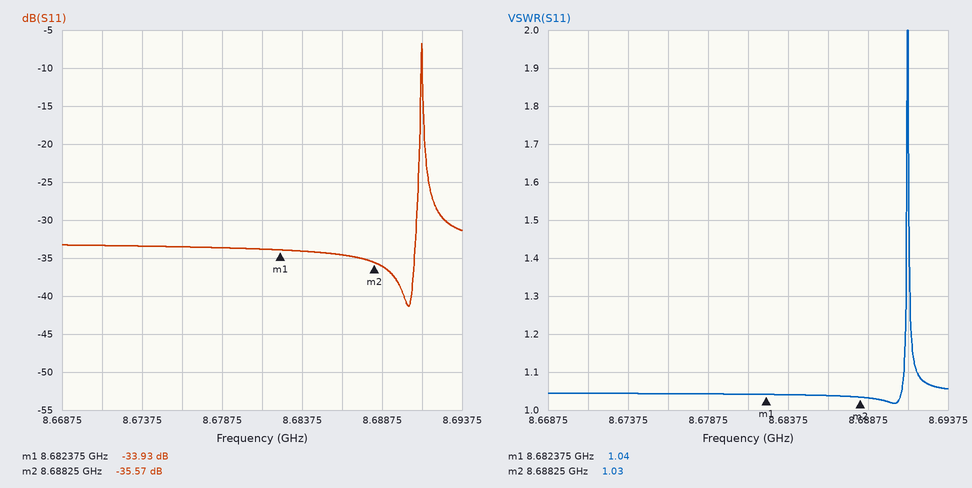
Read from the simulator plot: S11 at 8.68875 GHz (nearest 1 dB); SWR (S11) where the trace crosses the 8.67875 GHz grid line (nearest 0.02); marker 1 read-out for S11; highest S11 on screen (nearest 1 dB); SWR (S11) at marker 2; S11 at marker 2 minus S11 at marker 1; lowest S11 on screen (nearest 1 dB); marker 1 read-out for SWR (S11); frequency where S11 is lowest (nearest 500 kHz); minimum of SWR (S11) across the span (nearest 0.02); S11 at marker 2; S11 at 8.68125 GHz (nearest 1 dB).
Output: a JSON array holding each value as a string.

["-36 dB", "1.04", "-33.93 dB", "-7 dB", "1.03", "-1.64 dB", "-41 dB", "1.04", "8.6905 GHz", "1.02", "-35.57 dB", "-34 dB"]
